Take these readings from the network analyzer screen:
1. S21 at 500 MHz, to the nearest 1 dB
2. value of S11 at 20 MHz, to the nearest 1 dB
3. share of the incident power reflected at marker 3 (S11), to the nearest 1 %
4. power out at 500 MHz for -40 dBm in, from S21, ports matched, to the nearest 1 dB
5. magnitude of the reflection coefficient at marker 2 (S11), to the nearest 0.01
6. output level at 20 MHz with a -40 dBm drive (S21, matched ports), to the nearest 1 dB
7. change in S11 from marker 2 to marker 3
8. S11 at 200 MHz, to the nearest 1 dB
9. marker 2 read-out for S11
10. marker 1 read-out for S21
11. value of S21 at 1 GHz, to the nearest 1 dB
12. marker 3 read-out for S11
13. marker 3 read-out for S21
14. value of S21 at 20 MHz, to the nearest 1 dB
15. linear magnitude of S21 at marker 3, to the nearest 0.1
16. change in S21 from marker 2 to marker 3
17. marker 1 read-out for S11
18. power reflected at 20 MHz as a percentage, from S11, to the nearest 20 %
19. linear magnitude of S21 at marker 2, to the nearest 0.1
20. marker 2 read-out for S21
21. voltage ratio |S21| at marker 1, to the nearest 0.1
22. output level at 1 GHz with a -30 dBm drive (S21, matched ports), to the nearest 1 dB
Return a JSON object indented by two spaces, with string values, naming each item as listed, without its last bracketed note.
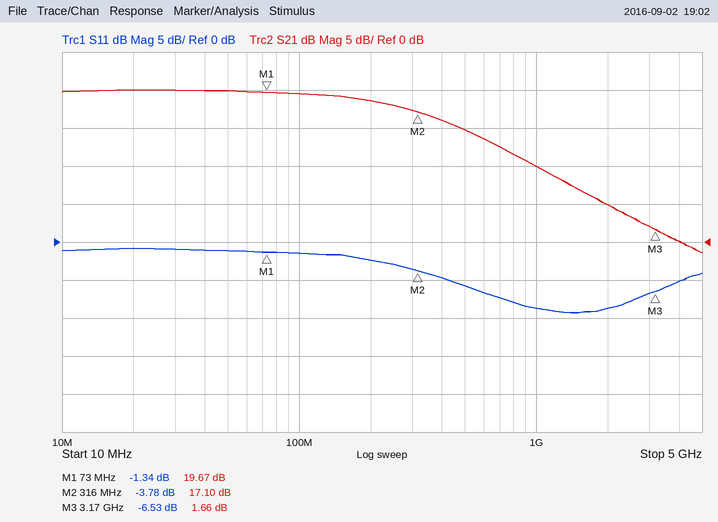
{
  "S21 at 500 MHz, to the nearest 1 dB": "15 dB",
  "value of S11 at 20 MHz, to the nearest 1 dB": "-1 dB",
  "share of the incident power reflected at marker 3 (S11), to the nearest 1 %": "22 %",
  "power out at 500 MHz for -40 dBm in, from S21, ports matched, to the nearest 1 dB": "-25 dBm",
  "magnitude of the reflection coefficient at marker 2 (S11), to the nearest 0.01": "0.65",
  "output level at 20 MHz with a -40 dBm drive (S21, matched ports), to the nearest 1 dB": "-20 dBm",
  "change in S11 from marker 2 to marker 3": "-2.75 dB",
  "S11 at 200 MHz, to the nearest 1 dB": "-2 dB",
  "marker 2 read-out for S11": "-3.78 dB",
  "marker 1 read-out for S21": "19.67 dB",
  "value of S21 at 1 GHz, to the nearest 1 dB": "10 dB",
  "marker 3 read-out for S11": "-6.53 dB",
  "marker 3 read-out for S21": "1.66 dB",
  "value of S21 at 20 MHz, to the nearest 1 dB": "20 dB",
  "linear magnitude of S21 at marker 3, to the nearest 0.1": "1.2",
  "change in S21 from marker 2 to marker 3": "-15.44 dB",
  "marker 1 read-out for S11": "-1.34 dB",
  "power reflected at 20 MHz as a percentage, from S11, to the nearest 20 %": "80 %",
  "linear magnitude of S21 at marker 2, to the nearest 0.1": "7.2",
  "marker 2 read-out for S21": "17.10 dB",
  "voltage ratio |S21| at marker 1, to the nearest 0.1": "9.6",
  "output level at 1 GHz with a -30 dBm drive (S21, matched ports), to the nearest 1 dB": "-20 dBm"
}
